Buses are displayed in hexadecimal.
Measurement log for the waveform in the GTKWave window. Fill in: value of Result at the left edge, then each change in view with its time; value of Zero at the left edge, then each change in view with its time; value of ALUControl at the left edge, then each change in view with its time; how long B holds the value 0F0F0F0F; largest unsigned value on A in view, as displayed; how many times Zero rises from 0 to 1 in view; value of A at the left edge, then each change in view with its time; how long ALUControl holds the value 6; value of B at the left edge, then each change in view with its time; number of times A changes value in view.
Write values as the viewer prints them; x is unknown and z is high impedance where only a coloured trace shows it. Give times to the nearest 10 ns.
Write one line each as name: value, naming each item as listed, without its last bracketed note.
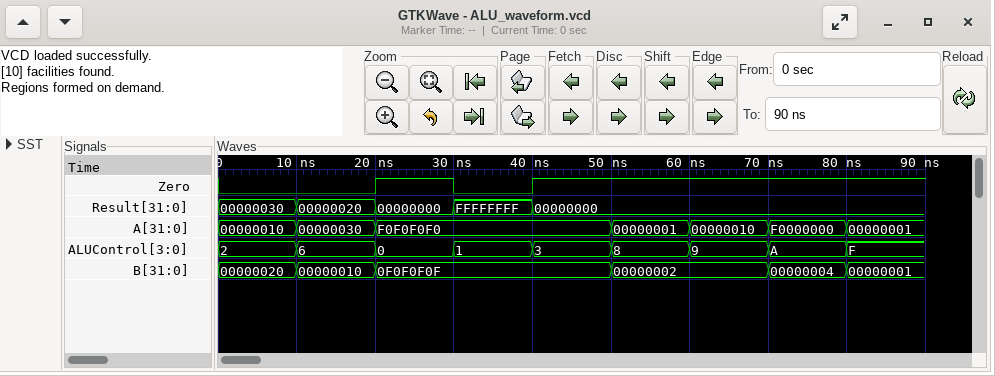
value of Result at the left edge, then each change in view with its time: 00000030, 00000020 at 10 ns, 00000000 at 20 ns, FFFFFFFF at 30 ns, 00000000 at 40 ns
value of Zero at the left edge, then each change in view with its time: 0, 1 at 20 ns, 0 at 30 ns, 1 at 40 ns
value of ALUControl at the left edge, then each change in view with its time: 2, 6 at 10 ns, 0 at 20 ns, 1 at 30 ns, 3 at 40 ns, 8 at 50 ns, 9 at 60 ns, A at 70 ns, F at 80 ns
how long B holds the value 0F0F0F0F: 30 ns
largest unsigned value on A in view, as displayed: F0F0F0F0
how many times Zero rises from 0 to 1 in view: 2
value of A at the left edge, then each change in view with its time: 00000010, 00000030 at 10 ns, F0F0F0F0 at 20 ns, 00000001 at 50 ns, 00000010 at 60 ns, F0000000 at 70 ns, 00000001 at 80 ns
how long ALUControl holds the value 6: 10 ns
value of B at the left edge, then each change in view with its time: 00000020, 00000010 at 10 ns, 0F0F0F0F at 20 ns, 00000002 at 50 ns, 00000004 at 70 ns, 00000001 at 80 ns
number of times A changes value in view: 6
